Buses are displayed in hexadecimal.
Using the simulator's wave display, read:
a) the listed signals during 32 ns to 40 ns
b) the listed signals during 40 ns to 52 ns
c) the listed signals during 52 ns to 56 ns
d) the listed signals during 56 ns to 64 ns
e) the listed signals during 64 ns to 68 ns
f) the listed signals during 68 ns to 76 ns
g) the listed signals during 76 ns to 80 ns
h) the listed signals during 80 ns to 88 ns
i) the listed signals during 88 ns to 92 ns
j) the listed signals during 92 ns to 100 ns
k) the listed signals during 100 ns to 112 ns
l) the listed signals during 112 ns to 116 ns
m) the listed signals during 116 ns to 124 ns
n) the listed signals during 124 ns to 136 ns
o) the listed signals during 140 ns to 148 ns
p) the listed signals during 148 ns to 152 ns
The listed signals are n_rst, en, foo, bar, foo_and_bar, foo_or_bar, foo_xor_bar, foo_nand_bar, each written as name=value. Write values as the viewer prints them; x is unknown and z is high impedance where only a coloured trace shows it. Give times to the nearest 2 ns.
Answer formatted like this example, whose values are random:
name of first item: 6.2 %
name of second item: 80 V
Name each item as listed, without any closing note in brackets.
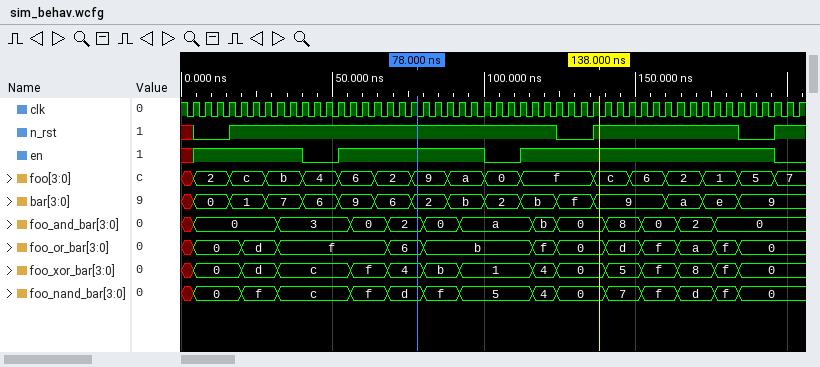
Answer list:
the listed signals during 32 ns to 40 ns: n_rst=1, en=1, foo=b, bar=7, foo_and_bar=3, foo_or_bar=f, foo_xor_bar=c, foo_nand_bar=c
the listed signals during 40 ns to 52 ns: n_rst=1, en=0, foo=4, bar=6, foo_and_bar=3, foo_or_bar=f, foo_xor_bar=c, foo_nand_bar=c
the listed signals during 52 ns to 56 ns: n_rst=1, en=1, foo=6, bar=9, foo_and_bar=3, foo_or_bar=f, foo_xor_bar=c, foo_nand_bar=c
the listed signals during 56 ns to 64 ns: n_rst=1, en=1, foo=6, bar=9, foo_and_bar=0, foo_or_bar=f, foo_xor_bar=f, foo_nand_bar=f
the listed signals during 64 ns to 68 ns: n_rst=1, en=1, foo=2, bar=6, foo_and_bar=0, foo_or_bar=f, foo_xor_bar=f, foo_nand_bar=f
the listed signals during 68 ns to 76 ns: n_rst=1, en=1, foo=2, bar=6, foo_and_bar=2, foo_or_bar=6, foo_xor_bar=4, foo_nand_bar=d
the listed signals during 76 ns to 80 ns: n_rst=1, en=1, foo=9, bar=2, foo_and_bar=2, foo_or_bar=6, foo_xor_bar=4, foo_nand_bar=d
the listed signals during 80 ns to 88 ns: n_rst=1, en=1, foo=9, bar=2, foo_and_bar=0, foo_or_bar=b, foo_xor_bar=b, foo_nand_bar=f
the listed signals during 88 ns to 92 ns: n_rst=1, en=1, foo=a, bar=b, foo_and_bar=0, foo_or_bar=b, foo_xor_bar=b, foo_nand_bar=f
the listed signals during 92 ns to 100 ns: n_rst=1, en=1, foo=a, bar=b, foo_and_bar=a, foo_or_bar=b, foo_xor_bar=1, foo_nand_bar=5
the listed signals during 100 ns to 112 ns: n_rst=1, en=0, foo=0, bar=2, foo_and_bar=a, foo_or_bar=b, foo_xor_bar=1, foo_nand_bar=5
the listed signals during 112 ns to 116 ns: n_rst=1, en=1, foo=f, bar=b, foo_and_bar=a, foo_or_bar=b, foo_xor_bar=1, foo_nand_bar=5
the listed signals during 116 ns to 124 ns: n_rst=1, en=1, foo=f, bar=b, foo_and_bar=b, foo_or_bar=f, foo_xor_bar=4, foo_nand_bar=4
the listed signals during 124 ns to 136 ns: n_rst=0, en=1, foo=f, bar=f, foo_and_bar=0, foo_or_bar=0, foo_xor_bar=0, foo_nand_bar=0
the listed signals during 140 ns to 148 ns: n_rst=1, en=1, foo=c, bar=9, foo_and_bar=8, foo_or_bar=d, foo_xor_bar=5, foo_nand_bar=7
the listed signals during 148 ns to 152 ns: n_rst=1, en=1, foo=6, bar=9, foo_and_bar=8, foo_or_bar=d, foo_xor_bar=5, foo_nand_bar=7
